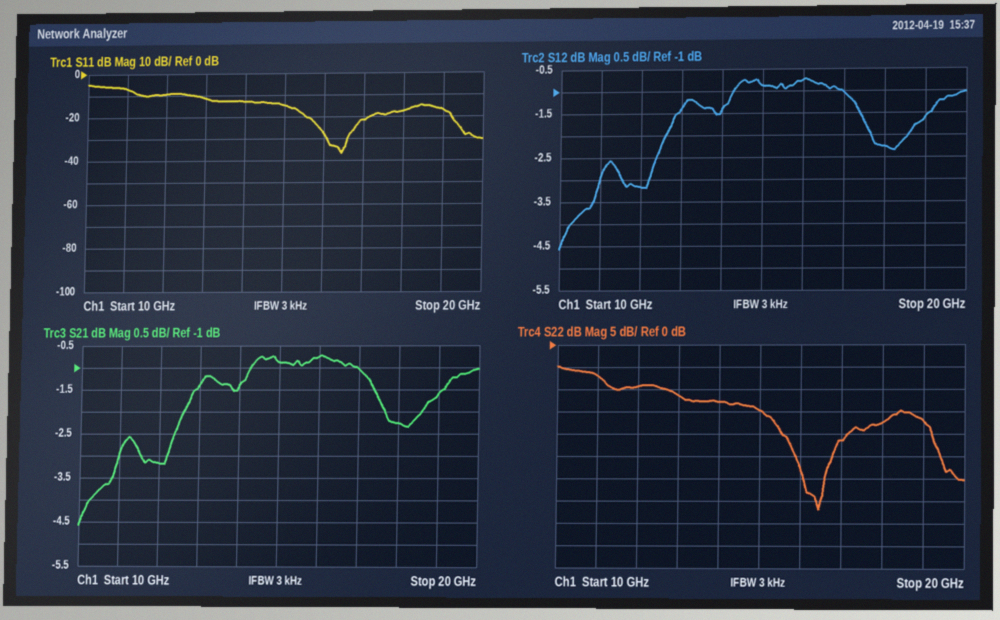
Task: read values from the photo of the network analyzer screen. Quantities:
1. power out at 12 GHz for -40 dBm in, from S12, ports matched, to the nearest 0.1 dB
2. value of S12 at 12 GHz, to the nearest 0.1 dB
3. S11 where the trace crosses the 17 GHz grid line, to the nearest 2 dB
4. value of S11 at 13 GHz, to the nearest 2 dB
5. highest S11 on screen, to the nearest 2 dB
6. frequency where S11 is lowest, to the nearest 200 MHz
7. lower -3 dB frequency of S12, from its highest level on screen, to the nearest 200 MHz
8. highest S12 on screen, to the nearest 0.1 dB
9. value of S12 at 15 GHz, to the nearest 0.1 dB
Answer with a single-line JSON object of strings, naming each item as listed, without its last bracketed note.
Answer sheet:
{"power out at 12 GHz for -40 dBm in, from S12, ports matched, to the nearest 0.1 dB": "-43.2 dBm", "value of S12 at 12 GHz, to the nearest 0.1 dB": "-3.2 dB", "S11 where the trace crosses the 17 GHz grid line, to the nearest 2 dB": "-22 dB", "value of S11 at 13 GHz, to the nearest 2 dB": "-12 dB", "highest S11 on screen, to the nearest 2 dB": "-4 dB", "frequency where S11 is lowest, to the nearest 200 MHz": "16.4 GHz", "lower -3 dB frequency of S12, from its highest level on screen, to the nearest 200 MHz": "10.6 GHz", "highest S12 on screen, to the nearest 0.1 dB": "-0.7 dB", "value of S12 at 15 GHz, to the nearest 0.1 dB": "-0.9 dB"}
